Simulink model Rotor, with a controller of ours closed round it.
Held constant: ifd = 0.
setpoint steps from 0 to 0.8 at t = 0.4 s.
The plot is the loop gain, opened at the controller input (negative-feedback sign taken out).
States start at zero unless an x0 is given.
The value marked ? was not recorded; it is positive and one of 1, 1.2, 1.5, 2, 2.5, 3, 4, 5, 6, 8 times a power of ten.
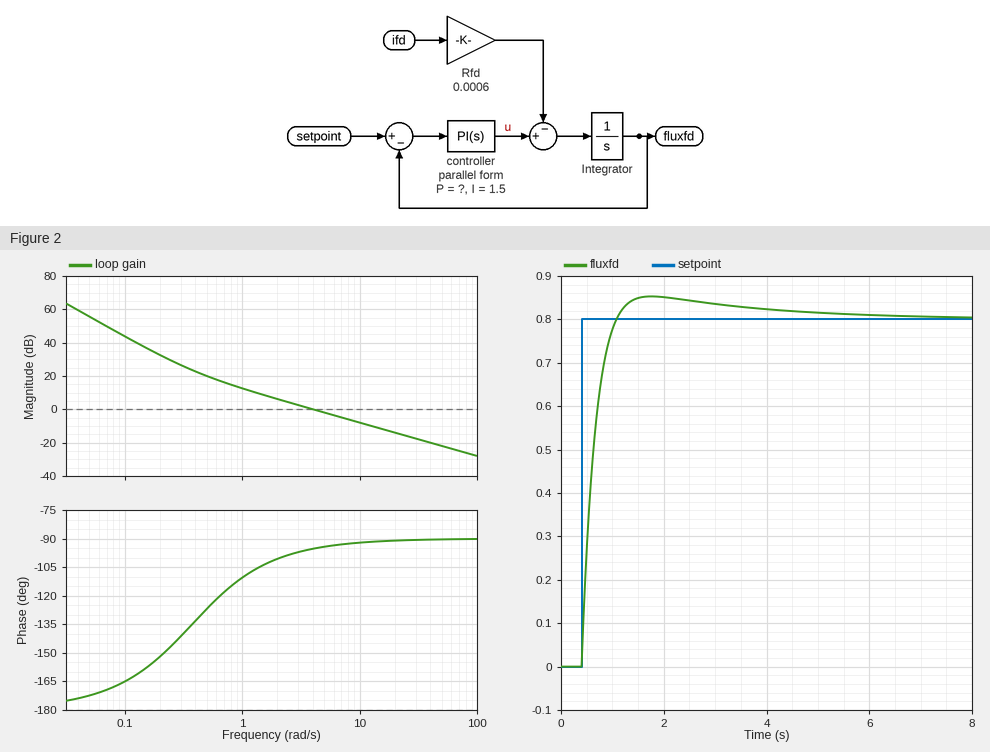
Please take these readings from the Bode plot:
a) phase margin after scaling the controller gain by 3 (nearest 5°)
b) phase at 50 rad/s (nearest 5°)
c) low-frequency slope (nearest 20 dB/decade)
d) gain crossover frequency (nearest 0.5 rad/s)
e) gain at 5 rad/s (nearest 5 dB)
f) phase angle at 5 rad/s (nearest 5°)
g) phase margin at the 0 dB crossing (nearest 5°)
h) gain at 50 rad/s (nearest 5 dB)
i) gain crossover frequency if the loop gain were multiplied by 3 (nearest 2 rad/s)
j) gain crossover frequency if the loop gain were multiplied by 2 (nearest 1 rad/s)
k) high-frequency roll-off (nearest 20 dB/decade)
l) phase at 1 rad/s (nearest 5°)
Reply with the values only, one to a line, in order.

90°
-90°
-40 dB/decade
4.0 rad/s
0 dB
-95°
85°
-20 dB
12 rad/s
8 rad/s
-20 dB/decade
-110°
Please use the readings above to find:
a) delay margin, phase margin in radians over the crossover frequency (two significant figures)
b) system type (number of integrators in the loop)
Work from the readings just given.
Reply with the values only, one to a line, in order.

0.37 s
2
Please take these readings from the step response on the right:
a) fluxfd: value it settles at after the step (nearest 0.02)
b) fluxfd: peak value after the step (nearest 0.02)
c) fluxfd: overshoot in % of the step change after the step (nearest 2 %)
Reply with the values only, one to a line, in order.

0.80
0.86
6 %
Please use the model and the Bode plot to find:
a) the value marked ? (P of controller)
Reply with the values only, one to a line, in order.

4
